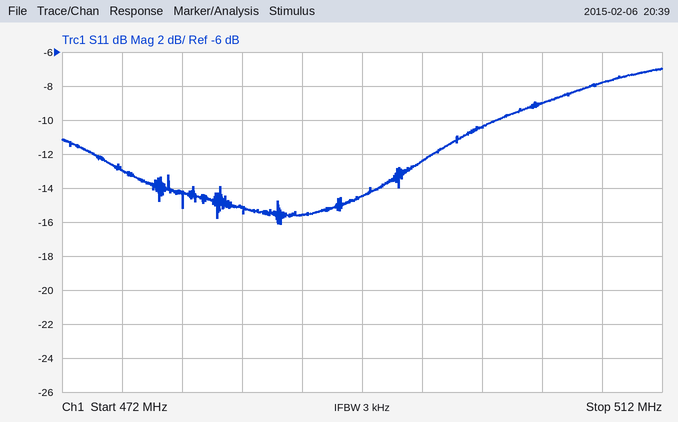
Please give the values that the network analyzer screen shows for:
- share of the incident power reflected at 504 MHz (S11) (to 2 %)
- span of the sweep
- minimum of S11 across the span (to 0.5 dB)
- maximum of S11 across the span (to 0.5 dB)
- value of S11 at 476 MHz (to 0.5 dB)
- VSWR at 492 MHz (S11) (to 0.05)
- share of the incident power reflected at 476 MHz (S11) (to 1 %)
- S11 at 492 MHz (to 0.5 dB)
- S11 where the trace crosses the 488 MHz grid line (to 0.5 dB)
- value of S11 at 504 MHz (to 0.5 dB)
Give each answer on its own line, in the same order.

12 %
40 MHz
-16.0 dB
-7.0 dB
-13.0 dB
1.45
5 %
-14.5 dB
-15.5 dB
-9.0 dB
